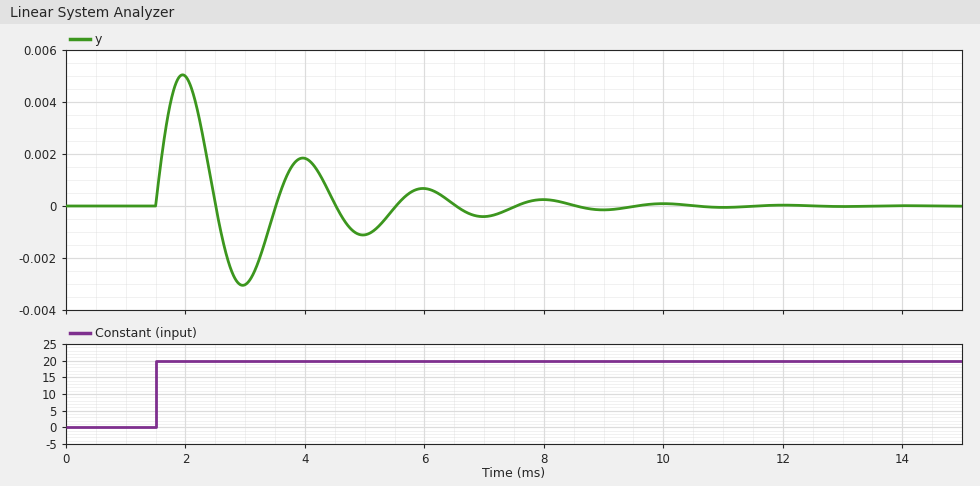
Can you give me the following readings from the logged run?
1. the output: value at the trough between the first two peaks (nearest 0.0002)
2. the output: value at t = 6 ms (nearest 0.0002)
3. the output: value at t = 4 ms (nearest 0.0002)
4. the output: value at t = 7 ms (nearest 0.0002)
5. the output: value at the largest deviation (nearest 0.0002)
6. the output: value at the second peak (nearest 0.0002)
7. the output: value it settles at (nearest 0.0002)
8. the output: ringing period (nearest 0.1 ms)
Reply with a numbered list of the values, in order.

1. -0.0030
2. 0.0006
3. 0.0018
4. -0.0004
5. 0.0050
6. 0.0018
7. 0.0000
8. 2.0 ms
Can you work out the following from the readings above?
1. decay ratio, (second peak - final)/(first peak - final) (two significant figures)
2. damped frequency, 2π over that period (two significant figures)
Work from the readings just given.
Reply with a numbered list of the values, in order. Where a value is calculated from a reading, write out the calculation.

1. (0.0018 - 0) / (0.005 - 0) = 0.36
2. 2π / 2 = 3.1 rad/ms
